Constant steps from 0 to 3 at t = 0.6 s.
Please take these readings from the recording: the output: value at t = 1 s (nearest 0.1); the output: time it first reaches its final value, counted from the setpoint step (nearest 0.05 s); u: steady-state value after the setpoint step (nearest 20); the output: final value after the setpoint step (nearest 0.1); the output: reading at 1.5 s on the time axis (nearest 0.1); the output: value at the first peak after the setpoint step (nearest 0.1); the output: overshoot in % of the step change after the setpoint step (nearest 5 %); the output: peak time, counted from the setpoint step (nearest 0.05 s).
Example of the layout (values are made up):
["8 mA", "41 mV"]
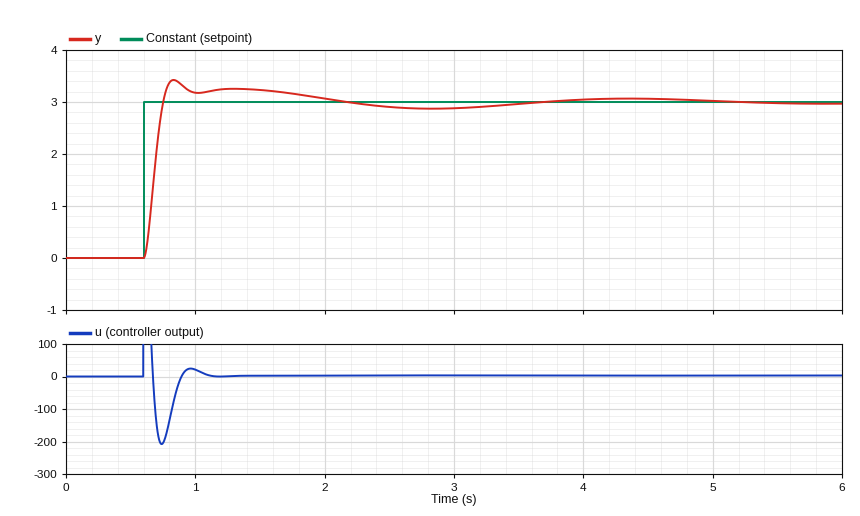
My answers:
["3.2", "0.15 s", "0", "3.0", "3.2", "3.4", "15 %", "0.25 s"]
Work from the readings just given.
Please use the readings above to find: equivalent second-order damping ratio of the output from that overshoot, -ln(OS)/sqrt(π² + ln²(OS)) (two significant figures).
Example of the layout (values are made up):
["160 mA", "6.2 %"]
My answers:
["0.52"]
